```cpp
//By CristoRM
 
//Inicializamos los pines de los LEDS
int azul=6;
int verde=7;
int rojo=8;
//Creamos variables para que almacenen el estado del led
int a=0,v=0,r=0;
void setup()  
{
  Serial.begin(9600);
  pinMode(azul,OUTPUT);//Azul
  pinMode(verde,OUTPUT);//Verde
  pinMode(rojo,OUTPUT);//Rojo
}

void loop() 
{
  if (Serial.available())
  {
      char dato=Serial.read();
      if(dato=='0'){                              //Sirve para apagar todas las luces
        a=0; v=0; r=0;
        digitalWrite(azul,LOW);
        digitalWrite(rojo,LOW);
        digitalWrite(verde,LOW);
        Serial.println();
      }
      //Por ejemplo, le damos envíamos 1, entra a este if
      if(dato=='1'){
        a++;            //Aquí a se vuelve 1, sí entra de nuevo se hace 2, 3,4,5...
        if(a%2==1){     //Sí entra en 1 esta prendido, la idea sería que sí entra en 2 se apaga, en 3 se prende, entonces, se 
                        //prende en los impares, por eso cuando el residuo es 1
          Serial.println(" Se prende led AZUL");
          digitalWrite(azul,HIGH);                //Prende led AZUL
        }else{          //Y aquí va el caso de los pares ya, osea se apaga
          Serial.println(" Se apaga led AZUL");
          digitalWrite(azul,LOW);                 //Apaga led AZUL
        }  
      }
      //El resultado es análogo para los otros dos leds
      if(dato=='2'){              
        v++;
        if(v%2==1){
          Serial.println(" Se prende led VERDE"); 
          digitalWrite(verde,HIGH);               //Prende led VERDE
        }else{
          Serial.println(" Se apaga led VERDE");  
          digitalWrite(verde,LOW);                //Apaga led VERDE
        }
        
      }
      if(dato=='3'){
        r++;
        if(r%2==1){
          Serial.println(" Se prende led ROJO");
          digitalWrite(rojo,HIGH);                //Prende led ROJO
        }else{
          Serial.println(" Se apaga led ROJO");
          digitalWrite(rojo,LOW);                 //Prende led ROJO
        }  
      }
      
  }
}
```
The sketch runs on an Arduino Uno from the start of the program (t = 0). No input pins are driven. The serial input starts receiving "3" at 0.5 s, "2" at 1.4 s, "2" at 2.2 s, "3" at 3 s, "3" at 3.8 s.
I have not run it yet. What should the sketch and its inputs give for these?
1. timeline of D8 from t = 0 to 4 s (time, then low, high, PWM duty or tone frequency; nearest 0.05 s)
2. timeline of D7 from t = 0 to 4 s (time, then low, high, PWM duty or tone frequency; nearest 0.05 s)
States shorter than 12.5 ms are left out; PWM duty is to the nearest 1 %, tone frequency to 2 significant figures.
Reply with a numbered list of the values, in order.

1. 0 s low; 0.5 s high; 3 s low; 3.8 s high
2. 0 s low; 1.4 s high; 2.2 s low
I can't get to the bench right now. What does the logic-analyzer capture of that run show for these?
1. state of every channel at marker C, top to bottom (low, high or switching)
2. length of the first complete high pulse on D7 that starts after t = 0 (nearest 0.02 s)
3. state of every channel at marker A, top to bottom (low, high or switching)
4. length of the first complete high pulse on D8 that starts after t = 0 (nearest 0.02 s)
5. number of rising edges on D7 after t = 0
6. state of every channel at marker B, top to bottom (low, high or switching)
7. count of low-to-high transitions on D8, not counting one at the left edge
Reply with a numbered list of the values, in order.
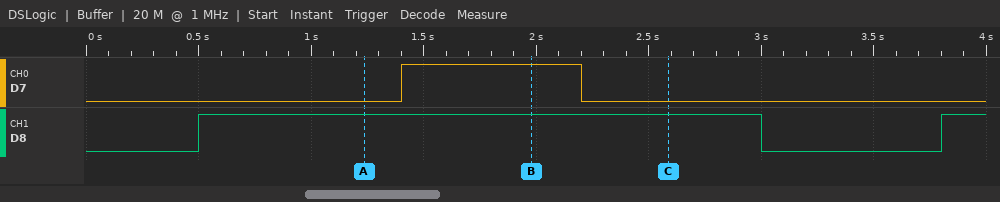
1. D7 low, D8 high
2. 0.80 s
3. D7 low, D8 high
4. 2.50 s
5. 1
6. D7 high, D8 high
7. 2
